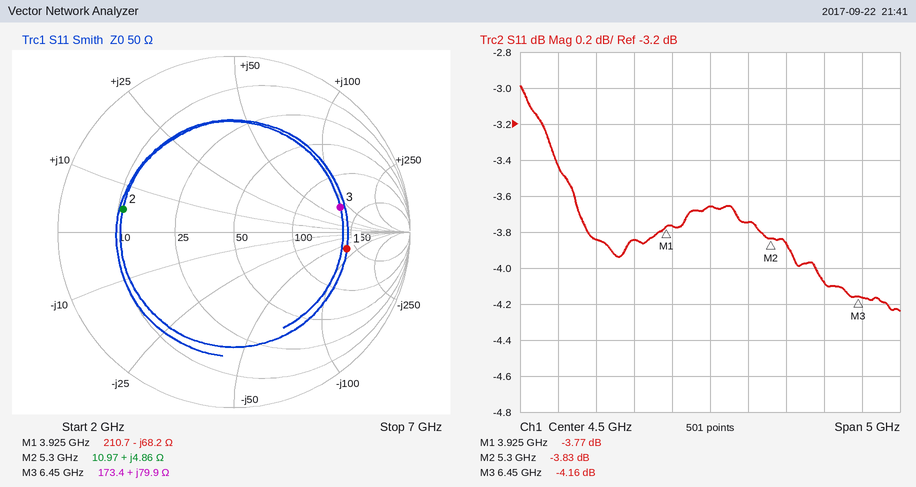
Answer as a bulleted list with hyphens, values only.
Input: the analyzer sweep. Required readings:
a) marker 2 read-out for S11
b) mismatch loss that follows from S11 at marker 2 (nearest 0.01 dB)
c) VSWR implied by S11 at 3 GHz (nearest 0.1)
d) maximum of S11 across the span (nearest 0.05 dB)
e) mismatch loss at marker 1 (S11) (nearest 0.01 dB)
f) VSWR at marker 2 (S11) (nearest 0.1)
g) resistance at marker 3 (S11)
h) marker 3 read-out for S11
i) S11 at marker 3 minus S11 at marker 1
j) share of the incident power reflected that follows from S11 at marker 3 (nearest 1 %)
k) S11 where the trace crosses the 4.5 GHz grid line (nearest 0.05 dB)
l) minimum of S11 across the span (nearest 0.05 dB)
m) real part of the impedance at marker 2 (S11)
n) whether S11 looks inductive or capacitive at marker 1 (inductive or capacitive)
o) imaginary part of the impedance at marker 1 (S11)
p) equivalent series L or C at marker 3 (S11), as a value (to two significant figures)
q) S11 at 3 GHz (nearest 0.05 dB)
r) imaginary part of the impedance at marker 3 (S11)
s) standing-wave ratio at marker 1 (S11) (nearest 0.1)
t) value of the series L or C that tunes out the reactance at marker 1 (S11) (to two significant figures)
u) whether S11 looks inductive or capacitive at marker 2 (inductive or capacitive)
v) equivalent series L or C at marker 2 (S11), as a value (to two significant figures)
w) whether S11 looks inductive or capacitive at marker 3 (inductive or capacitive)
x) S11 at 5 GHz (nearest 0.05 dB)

- -3.83 dB
- 2.32 dB
- 4.6
- -3.00 dB
- 2.36 dB
- 4.6
- 173.4 Ω
- -4.16 dB
- -0.39 dB
- 38 %
- -3.65 dB
- -4.25 dB
- 10.97 Ω
- capacitive
- -68.2 Ω
- 2.0 nH
- -3.85 dB
- +79.9 Ω
- 4.7
- 2.8 nH
- inductive
- 150 pH
- inductive
- -3.75 dB
